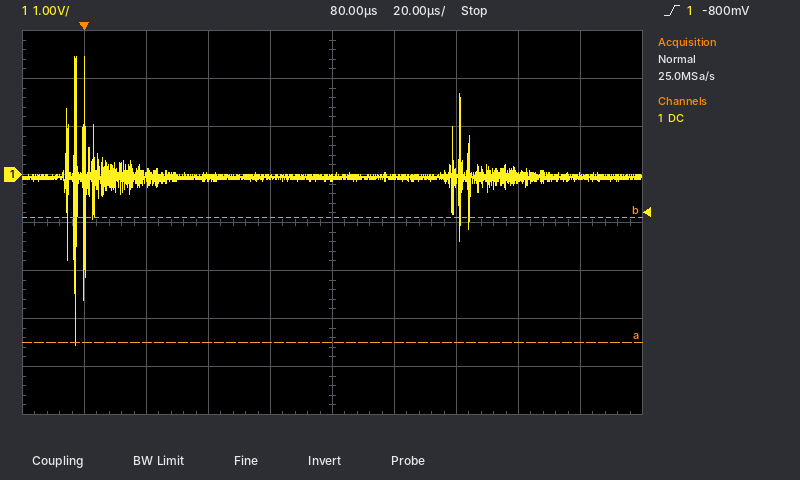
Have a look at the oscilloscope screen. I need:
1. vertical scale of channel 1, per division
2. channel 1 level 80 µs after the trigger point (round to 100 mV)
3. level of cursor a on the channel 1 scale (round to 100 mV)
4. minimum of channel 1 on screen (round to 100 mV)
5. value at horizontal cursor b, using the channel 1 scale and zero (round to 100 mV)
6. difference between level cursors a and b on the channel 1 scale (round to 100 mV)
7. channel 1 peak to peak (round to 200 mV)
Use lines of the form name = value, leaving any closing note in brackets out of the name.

vertical scale of channel 1, per division = 1 V
channel 1 level 80 µs after the trigger point = -100 mV
level of cursor a on the channel 1 scale = -3.5 V
minimum of channel 1 on screen = -3.5 V
value at horizontal cursor b, using the channel 1 scale and zero = -900 mV
difference between level cursors a and b on the channel 1 scale = 2.6 V
channel 1 peak to peak = 6.0 V
